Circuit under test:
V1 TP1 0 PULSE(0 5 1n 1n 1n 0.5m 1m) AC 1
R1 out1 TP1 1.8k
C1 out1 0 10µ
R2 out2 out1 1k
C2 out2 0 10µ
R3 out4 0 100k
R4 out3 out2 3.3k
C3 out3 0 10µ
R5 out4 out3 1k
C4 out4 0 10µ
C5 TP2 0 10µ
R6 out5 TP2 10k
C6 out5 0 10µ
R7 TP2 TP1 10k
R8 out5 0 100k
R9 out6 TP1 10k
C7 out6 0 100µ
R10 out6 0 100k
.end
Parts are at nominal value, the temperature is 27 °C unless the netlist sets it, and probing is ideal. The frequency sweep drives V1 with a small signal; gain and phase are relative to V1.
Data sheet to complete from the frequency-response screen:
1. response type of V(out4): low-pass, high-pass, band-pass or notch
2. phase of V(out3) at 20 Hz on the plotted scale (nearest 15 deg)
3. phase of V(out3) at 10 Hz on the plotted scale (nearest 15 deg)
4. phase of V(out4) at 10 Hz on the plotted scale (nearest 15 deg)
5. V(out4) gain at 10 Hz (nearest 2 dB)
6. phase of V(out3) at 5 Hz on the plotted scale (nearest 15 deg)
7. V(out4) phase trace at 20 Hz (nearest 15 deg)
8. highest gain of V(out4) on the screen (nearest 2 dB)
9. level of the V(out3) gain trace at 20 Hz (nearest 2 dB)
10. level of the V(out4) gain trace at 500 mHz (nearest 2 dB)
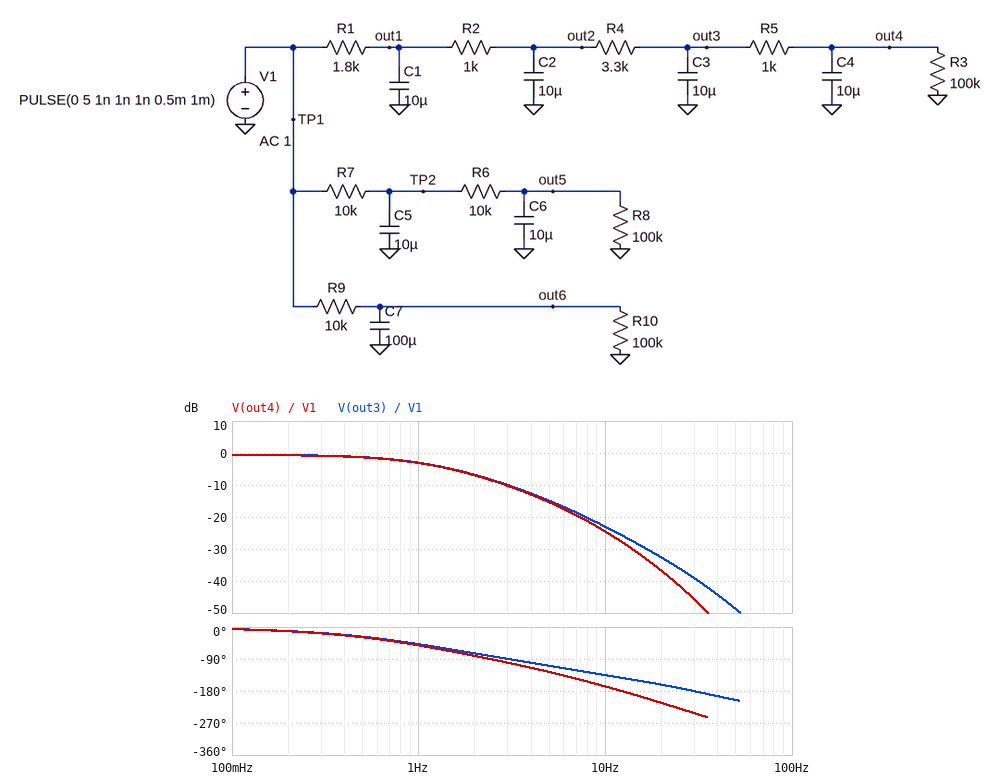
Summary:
low-pass
-165 deg
-135 deg
-165 deg
-24 dB
-105 deg
-210 deg
0 dB
-32 dB
-2 dB
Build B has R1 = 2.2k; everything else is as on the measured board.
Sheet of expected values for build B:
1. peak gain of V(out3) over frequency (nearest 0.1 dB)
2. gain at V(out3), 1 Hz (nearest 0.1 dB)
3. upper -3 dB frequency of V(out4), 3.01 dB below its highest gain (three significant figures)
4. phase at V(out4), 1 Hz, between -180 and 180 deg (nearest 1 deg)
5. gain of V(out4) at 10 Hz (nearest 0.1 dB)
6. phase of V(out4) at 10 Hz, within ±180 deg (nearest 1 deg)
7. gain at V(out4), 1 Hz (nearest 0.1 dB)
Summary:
-0.5 dB
-3.4 dB
1.03 Hz
-55 deg
-25.8 dB
-170 deg
-3.5 dB
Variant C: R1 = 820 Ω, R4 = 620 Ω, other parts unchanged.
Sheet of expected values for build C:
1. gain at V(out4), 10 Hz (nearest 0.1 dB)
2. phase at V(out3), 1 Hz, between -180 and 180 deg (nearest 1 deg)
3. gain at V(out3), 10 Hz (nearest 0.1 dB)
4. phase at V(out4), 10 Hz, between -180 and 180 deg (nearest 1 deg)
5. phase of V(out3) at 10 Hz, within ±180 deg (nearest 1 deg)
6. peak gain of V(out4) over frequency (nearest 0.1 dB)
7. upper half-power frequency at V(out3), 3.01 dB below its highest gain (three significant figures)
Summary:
-14.6 dB
-25 deg
-13.1 dB
-126 deg
-94 deg
-0.3 dB
2.32 Hz
